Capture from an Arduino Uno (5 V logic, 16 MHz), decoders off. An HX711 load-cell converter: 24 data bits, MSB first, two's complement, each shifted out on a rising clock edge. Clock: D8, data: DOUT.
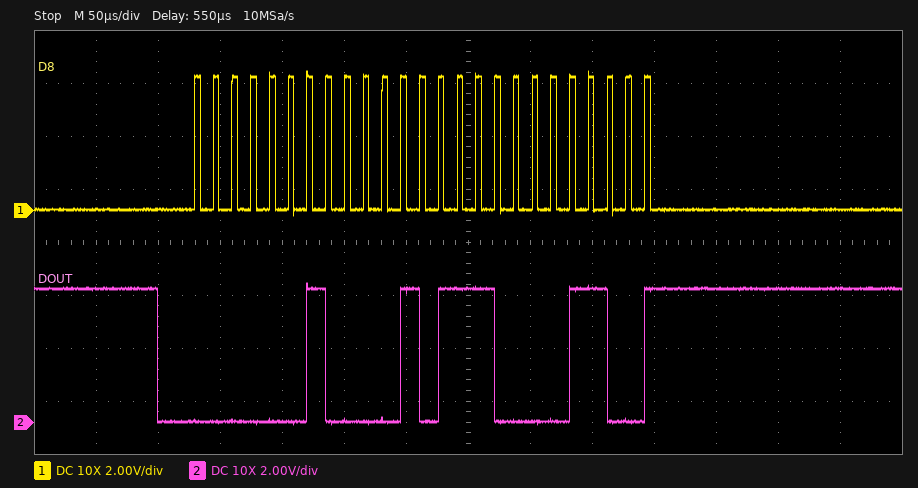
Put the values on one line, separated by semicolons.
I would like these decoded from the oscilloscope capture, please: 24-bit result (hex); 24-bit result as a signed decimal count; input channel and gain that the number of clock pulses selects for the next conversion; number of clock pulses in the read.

0x02170C; 136972; channel A, gain 128; 25
